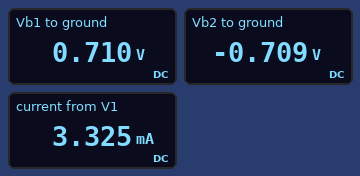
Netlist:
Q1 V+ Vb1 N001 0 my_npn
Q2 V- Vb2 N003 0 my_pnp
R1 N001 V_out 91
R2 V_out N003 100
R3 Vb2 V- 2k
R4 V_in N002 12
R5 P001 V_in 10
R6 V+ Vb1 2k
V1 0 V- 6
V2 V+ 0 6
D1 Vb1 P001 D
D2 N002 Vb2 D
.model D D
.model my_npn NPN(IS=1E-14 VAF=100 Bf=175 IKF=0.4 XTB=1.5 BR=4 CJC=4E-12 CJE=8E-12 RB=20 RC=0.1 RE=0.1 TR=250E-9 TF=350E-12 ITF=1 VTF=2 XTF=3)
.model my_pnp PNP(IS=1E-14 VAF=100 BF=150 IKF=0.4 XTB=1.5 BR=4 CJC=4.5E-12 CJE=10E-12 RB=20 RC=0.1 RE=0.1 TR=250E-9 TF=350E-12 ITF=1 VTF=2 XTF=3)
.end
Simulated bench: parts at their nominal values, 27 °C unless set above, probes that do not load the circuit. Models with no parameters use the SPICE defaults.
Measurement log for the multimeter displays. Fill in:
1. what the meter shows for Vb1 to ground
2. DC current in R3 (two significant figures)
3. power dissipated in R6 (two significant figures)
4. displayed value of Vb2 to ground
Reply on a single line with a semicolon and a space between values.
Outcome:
0.710 V; 2.6 mA; 14 mW; -0.709 V
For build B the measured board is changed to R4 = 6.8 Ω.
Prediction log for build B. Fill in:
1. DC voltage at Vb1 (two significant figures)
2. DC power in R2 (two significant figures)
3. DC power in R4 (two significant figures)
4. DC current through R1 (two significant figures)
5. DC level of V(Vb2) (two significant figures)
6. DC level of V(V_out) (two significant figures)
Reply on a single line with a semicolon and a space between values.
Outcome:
700 mV; 40 µW; 48 µW; 630 µA; -700 mV; 3.4 mV
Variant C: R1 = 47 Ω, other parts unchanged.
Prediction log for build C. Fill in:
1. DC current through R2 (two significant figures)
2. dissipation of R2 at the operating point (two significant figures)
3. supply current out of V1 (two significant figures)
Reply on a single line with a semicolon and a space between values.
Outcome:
820 µA; 68 µW; 3.5 mA
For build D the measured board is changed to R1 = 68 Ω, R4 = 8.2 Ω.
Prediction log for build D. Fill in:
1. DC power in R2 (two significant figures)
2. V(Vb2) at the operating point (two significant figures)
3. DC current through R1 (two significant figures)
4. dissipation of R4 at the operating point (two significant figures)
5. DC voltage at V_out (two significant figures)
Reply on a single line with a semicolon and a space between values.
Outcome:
50 µW; -700 mV; 710 µA; 57 µW; 12 mV
